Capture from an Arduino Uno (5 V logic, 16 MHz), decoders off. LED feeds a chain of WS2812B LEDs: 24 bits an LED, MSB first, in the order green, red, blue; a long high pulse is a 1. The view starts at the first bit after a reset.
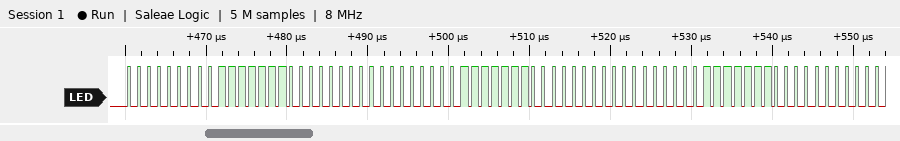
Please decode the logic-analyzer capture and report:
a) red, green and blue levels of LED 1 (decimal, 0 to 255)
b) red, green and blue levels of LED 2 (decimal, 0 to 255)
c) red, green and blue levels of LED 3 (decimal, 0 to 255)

127, 0, 0
127, 0, 0
127, 0, 0
